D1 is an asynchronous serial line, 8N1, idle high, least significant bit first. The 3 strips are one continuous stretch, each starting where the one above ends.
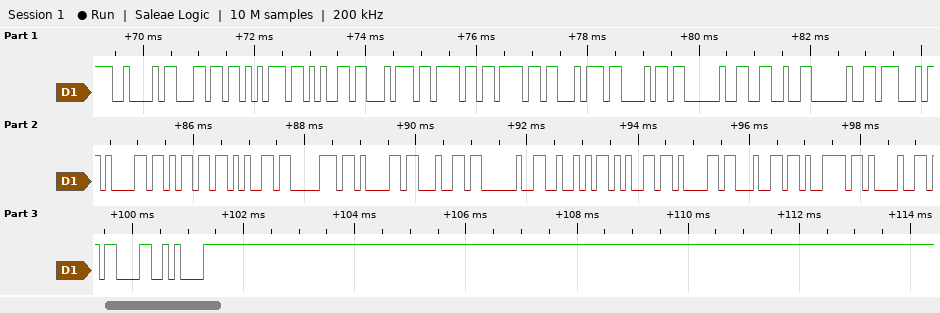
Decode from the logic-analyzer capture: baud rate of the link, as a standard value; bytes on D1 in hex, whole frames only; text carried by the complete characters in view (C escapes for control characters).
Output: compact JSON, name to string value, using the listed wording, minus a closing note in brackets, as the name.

{"baud rate of the link, as a standard value": "9600 baud", "bytes on D1 in hex, whole frames only": "42 6C 75 65 74 6F 6F 74 68 20 26 20 47 61 6D 65 70 61 64 20 52 65 61 64 79 21 0D 0A", "text carried by the complete characters in view": "\"Bluetooth & Gamepad Ready!\\r\\n\""}
